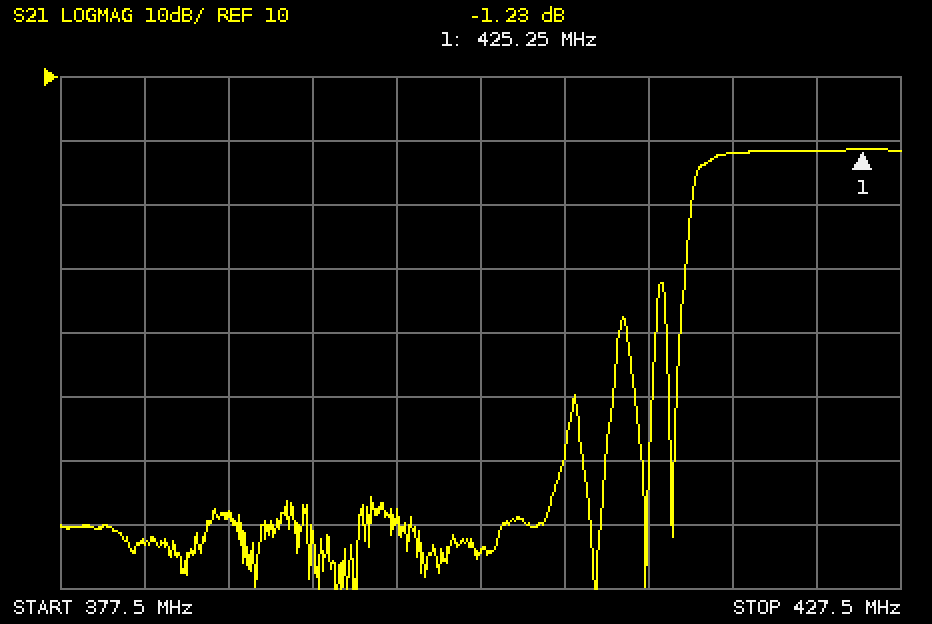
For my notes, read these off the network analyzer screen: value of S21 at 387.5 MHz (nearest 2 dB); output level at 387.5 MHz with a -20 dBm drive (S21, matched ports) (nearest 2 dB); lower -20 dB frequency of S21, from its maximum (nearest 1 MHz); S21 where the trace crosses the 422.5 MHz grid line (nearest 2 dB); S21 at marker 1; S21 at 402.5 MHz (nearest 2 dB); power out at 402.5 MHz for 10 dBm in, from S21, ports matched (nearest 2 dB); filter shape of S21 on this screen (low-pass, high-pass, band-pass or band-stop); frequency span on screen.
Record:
-58 dB
-78 dBm
415 MHz
-2 dB
-1.23 dB
-64 dB
-54 dBm
high-pass
50 MHz
